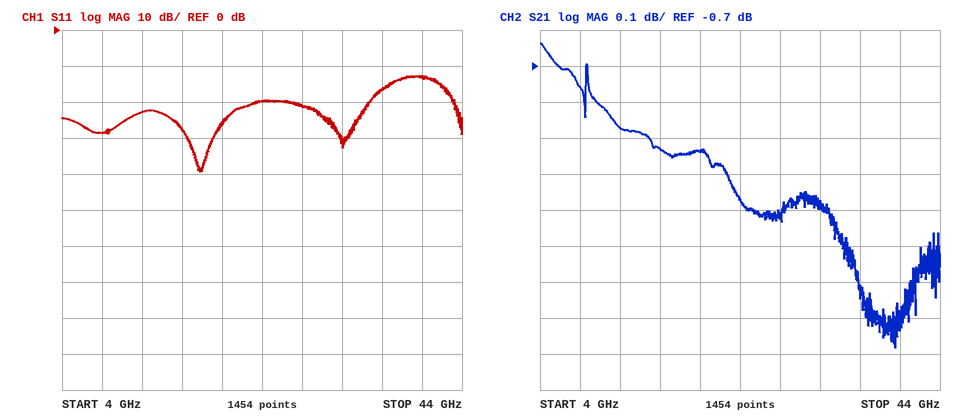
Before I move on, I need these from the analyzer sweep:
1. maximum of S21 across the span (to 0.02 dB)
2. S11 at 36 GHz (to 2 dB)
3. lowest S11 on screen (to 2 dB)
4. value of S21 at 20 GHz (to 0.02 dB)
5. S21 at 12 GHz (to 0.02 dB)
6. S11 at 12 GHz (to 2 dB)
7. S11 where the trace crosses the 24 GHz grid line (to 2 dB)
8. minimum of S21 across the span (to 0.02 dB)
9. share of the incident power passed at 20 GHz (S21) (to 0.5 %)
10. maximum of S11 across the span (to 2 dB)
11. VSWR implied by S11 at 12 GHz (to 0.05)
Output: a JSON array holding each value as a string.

["-0.64 dB", "-16 dB", "-40 dB", "-0.94 dB", "-0.88 dB", "-22 dB", "-20 dB", "-1.48 dB", "80.5 %", "-12 dB", "1.15"]
